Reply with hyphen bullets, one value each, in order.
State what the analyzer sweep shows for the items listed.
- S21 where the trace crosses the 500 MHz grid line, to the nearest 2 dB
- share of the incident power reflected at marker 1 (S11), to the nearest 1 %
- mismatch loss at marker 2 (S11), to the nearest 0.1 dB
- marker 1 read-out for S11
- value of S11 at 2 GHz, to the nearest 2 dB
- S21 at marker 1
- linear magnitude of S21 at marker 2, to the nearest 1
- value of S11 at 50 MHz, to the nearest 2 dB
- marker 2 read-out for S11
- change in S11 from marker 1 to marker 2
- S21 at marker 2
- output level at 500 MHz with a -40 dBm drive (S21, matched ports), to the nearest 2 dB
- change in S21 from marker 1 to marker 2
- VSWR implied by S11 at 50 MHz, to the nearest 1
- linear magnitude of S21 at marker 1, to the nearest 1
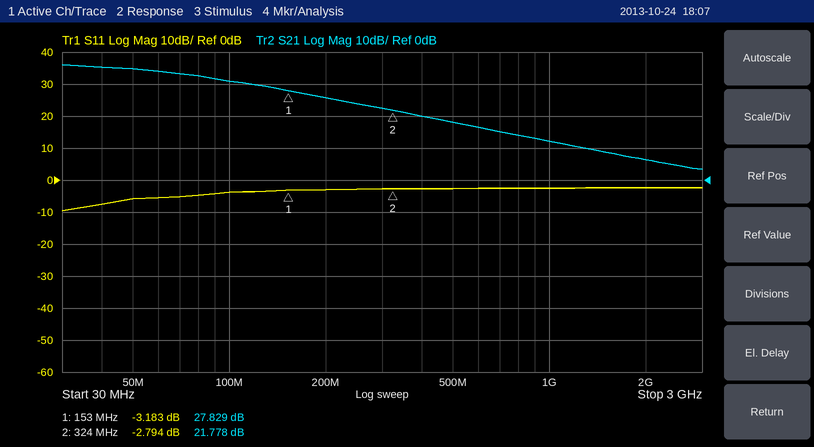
- 18 dB
- 48 %
- 3.2 dB
- -3.183 dB
- -2 dB
- 27.829 dB
- 12
- -6 dB
- -2.794 dB
- 0.389 dB
- 21.778 dB
- -22 dBm
- -6.051 dB
- 3
- 25
